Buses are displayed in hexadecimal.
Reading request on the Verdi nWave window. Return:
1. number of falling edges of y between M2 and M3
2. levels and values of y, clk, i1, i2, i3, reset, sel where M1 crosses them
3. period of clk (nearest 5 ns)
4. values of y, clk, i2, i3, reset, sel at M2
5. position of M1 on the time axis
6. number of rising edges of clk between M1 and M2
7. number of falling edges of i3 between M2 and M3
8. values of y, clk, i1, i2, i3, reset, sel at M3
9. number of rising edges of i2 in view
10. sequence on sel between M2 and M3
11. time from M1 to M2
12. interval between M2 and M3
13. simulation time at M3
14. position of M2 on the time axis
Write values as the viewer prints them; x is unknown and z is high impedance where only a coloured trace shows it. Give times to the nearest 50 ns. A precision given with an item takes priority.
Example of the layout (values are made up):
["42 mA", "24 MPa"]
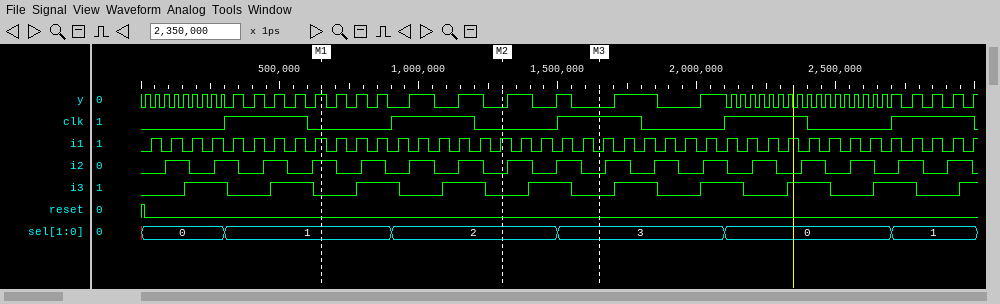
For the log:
["2", "y=1, clk=0, i1=1, i2=1, i3=0, reset=0, sel=1", "600 ns", "y=0, clk=0, i2=0, i3=0, reset=0, sel=2", "650 ns", "1", "1", "y=0, clk=1, i1=0, i2=0, i3=0, reset=0, sel=3", "17", "2, 3", "650 ns", "350 ns", "1650 ns", "1300 ns"]
